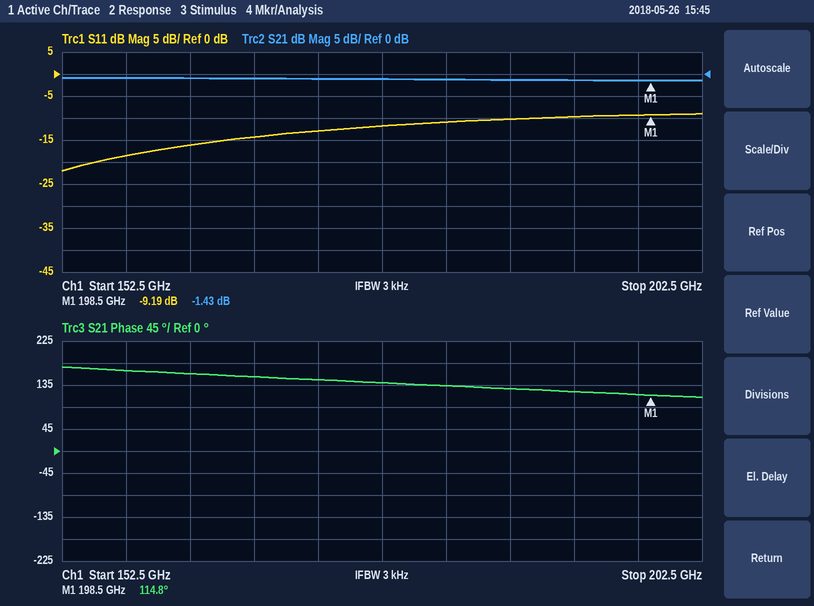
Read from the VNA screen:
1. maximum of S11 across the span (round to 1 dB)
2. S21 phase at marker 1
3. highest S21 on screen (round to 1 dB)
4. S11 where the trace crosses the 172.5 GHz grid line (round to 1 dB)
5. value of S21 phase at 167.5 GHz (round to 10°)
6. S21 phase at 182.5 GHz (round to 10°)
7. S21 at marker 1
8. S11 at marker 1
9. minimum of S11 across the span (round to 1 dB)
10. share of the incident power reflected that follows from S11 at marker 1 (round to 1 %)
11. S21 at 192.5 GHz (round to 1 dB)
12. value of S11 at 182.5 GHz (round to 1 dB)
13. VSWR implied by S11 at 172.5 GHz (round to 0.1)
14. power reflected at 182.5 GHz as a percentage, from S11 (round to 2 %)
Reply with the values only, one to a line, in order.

-9 dB
114.8°
-1 dB
-13 dB
150°
130°
-1.43 dB
-9.19 dB
-22 dB
12 %
-1 dB
-11 dB
1.6
8 %
